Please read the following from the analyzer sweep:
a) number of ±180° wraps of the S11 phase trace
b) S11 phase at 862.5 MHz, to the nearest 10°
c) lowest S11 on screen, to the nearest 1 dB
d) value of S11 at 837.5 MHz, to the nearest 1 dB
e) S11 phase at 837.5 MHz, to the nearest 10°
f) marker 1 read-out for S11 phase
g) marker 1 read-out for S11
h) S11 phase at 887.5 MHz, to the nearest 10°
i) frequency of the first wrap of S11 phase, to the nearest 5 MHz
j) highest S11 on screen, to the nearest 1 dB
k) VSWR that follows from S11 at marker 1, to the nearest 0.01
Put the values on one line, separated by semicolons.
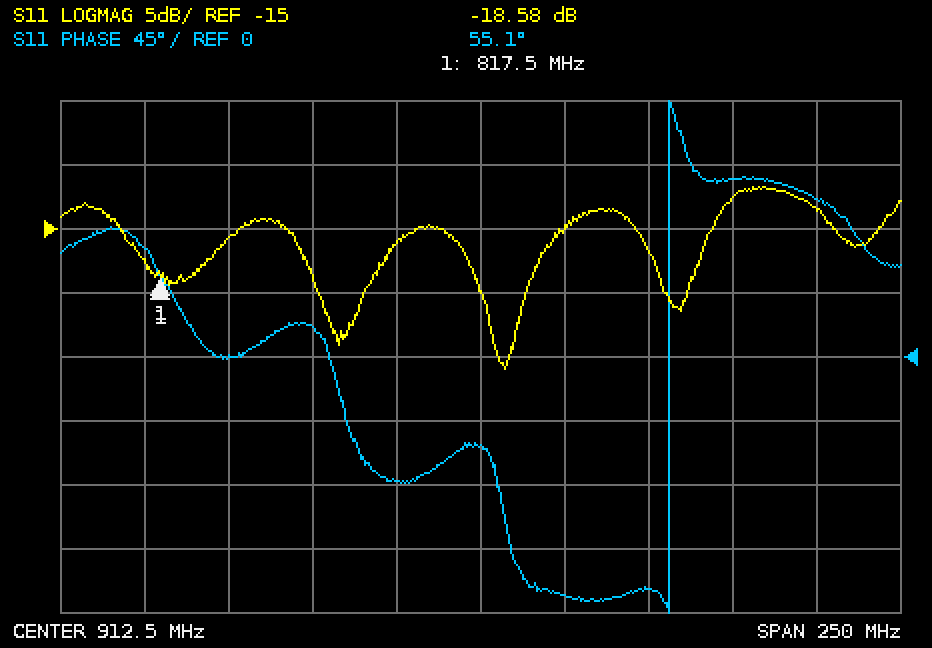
1; 20°; -26 dB; -16 dB; 0°; 55.1°; -18.58 dB; -90°; 970 MHz; -12 dB; 1.27
